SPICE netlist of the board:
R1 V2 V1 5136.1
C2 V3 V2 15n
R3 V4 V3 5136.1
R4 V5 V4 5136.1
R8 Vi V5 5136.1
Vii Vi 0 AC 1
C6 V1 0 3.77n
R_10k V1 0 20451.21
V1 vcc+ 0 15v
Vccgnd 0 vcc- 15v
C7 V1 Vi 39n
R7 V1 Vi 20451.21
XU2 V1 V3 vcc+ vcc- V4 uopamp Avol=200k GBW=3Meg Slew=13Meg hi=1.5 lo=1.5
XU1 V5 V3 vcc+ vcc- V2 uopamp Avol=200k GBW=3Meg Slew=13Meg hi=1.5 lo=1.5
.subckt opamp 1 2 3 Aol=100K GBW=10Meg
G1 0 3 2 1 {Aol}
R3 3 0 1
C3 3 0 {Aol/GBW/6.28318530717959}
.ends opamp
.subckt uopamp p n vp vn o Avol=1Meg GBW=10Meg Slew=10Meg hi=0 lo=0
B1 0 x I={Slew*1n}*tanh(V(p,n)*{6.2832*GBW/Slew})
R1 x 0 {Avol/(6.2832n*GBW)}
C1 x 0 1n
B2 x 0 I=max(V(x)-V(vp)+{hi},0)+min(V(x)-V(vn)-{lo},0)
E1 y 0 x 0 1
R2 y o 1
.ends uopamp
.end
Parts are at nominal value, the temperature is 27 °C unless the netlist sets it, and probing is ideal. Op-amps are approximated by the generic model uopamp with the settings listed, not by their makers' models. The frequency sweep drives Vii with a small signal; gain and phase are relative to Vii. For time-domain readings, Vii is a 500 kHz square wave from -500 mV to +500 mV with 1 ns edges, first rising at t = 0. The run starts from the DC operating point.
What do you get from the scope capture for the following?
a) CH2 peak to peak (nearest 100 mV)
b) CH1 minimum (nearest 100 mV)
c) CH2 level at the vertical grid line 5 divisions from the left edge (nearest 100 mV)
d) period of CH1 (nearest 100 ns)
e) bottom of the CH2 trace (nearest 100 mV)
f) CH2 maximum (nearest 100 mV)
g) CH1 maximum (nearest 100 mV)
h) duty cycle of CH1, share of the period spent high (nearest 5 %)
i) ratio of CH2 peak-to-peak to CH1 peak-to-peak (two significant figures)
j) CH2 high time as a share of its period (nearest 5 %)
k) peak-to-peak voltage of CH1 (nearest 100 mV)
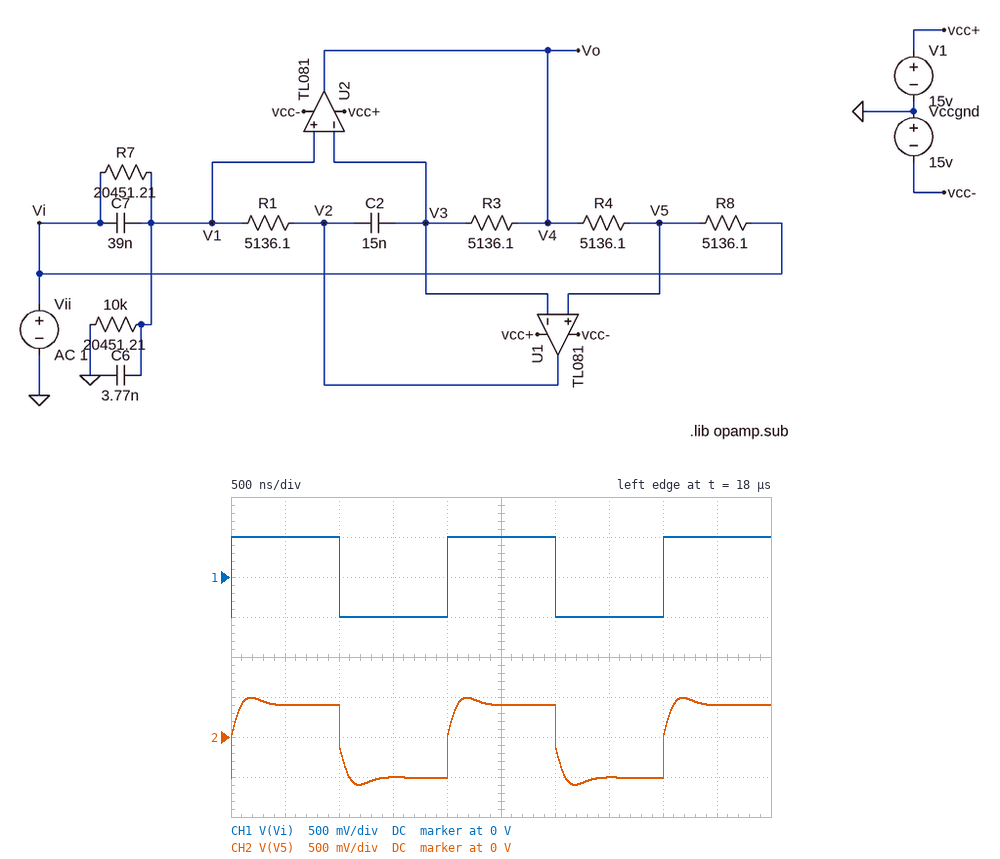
1.1 V
-500 mV
400 mV
2.0 µs
-600 mV
500 mV
500 mV
50 %
1.1
50 %
1.0 V
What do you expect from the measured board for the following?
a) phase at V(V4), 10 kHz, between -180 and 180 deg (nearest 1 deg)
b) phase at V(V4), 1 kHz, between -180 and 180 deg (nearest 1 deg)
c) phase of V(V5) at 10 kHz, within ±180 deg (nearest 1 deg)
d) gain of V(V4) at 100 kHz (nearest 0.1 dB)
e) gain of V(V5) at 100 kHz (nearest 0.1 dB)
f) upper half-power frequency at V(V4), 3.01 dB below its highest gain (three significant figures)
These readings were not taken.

2 deg
-36 deg
1 deg
-1.7 dB
-0.8 dB
3.50 MHz
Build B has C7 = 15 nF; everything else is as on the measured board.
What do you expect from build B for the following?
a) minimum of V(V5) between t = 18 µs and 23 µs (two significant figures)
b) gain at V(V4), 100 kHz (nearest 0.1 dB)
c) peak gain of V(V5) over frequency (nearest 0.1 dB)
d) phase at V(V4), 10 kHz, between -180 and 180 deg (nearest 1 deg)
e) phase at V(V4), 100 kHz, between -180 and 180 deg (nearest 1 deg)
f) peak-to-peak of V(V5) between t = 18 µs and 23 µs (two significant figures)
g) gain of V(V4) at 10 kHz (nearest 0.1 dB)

-610 mV
-4.4 dB
0.4 dB
5 deg
2 deg
1.0 V
-4.7 dB
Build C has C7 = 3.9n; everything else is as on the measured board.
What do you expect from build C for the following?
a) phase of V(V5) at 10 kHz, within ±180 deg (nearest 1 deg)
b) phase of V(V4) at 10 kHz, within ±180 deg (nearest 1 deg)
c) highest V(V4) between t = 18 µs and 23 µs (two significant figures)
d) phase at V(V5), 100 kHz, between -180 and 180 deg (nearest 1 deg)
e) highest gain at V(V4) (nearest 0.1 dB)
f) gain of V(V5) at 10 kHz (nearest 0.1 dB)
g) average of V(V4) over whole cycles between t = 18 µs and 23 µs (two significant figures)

-1 deg
-171 deg
-120 mV
2 deg
3.5 dB
-6.6 dB
-460 mV
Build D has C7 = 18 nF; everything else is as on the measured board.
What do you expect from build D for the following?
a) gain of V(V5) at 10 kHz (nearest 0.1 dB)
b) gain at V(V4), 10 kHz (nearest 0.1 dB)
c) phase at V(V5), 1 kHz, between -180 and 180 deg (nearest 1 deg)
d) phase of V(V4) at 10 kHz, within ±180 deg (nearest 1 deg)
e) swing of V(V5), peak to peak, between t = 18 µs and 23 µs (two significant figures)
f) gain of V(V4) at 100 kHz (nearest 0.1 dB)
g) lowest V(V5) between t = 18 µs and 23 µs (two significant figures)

-1.7 dB
-3.9 dB
-11 deg
4 deg
1.0 V
-3.7 dB
-610 mV
